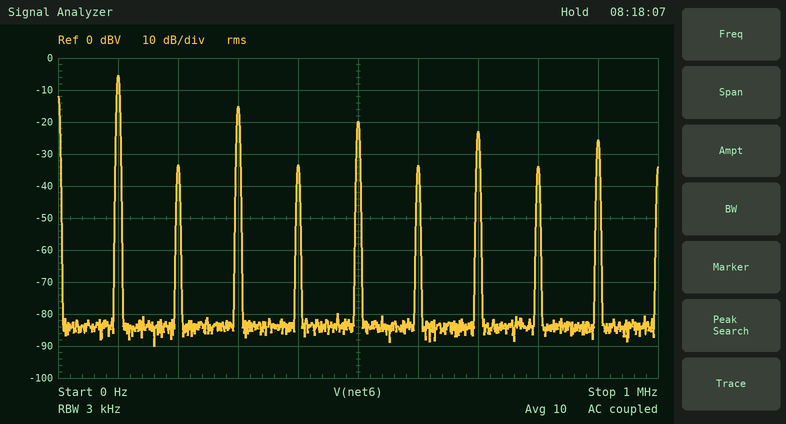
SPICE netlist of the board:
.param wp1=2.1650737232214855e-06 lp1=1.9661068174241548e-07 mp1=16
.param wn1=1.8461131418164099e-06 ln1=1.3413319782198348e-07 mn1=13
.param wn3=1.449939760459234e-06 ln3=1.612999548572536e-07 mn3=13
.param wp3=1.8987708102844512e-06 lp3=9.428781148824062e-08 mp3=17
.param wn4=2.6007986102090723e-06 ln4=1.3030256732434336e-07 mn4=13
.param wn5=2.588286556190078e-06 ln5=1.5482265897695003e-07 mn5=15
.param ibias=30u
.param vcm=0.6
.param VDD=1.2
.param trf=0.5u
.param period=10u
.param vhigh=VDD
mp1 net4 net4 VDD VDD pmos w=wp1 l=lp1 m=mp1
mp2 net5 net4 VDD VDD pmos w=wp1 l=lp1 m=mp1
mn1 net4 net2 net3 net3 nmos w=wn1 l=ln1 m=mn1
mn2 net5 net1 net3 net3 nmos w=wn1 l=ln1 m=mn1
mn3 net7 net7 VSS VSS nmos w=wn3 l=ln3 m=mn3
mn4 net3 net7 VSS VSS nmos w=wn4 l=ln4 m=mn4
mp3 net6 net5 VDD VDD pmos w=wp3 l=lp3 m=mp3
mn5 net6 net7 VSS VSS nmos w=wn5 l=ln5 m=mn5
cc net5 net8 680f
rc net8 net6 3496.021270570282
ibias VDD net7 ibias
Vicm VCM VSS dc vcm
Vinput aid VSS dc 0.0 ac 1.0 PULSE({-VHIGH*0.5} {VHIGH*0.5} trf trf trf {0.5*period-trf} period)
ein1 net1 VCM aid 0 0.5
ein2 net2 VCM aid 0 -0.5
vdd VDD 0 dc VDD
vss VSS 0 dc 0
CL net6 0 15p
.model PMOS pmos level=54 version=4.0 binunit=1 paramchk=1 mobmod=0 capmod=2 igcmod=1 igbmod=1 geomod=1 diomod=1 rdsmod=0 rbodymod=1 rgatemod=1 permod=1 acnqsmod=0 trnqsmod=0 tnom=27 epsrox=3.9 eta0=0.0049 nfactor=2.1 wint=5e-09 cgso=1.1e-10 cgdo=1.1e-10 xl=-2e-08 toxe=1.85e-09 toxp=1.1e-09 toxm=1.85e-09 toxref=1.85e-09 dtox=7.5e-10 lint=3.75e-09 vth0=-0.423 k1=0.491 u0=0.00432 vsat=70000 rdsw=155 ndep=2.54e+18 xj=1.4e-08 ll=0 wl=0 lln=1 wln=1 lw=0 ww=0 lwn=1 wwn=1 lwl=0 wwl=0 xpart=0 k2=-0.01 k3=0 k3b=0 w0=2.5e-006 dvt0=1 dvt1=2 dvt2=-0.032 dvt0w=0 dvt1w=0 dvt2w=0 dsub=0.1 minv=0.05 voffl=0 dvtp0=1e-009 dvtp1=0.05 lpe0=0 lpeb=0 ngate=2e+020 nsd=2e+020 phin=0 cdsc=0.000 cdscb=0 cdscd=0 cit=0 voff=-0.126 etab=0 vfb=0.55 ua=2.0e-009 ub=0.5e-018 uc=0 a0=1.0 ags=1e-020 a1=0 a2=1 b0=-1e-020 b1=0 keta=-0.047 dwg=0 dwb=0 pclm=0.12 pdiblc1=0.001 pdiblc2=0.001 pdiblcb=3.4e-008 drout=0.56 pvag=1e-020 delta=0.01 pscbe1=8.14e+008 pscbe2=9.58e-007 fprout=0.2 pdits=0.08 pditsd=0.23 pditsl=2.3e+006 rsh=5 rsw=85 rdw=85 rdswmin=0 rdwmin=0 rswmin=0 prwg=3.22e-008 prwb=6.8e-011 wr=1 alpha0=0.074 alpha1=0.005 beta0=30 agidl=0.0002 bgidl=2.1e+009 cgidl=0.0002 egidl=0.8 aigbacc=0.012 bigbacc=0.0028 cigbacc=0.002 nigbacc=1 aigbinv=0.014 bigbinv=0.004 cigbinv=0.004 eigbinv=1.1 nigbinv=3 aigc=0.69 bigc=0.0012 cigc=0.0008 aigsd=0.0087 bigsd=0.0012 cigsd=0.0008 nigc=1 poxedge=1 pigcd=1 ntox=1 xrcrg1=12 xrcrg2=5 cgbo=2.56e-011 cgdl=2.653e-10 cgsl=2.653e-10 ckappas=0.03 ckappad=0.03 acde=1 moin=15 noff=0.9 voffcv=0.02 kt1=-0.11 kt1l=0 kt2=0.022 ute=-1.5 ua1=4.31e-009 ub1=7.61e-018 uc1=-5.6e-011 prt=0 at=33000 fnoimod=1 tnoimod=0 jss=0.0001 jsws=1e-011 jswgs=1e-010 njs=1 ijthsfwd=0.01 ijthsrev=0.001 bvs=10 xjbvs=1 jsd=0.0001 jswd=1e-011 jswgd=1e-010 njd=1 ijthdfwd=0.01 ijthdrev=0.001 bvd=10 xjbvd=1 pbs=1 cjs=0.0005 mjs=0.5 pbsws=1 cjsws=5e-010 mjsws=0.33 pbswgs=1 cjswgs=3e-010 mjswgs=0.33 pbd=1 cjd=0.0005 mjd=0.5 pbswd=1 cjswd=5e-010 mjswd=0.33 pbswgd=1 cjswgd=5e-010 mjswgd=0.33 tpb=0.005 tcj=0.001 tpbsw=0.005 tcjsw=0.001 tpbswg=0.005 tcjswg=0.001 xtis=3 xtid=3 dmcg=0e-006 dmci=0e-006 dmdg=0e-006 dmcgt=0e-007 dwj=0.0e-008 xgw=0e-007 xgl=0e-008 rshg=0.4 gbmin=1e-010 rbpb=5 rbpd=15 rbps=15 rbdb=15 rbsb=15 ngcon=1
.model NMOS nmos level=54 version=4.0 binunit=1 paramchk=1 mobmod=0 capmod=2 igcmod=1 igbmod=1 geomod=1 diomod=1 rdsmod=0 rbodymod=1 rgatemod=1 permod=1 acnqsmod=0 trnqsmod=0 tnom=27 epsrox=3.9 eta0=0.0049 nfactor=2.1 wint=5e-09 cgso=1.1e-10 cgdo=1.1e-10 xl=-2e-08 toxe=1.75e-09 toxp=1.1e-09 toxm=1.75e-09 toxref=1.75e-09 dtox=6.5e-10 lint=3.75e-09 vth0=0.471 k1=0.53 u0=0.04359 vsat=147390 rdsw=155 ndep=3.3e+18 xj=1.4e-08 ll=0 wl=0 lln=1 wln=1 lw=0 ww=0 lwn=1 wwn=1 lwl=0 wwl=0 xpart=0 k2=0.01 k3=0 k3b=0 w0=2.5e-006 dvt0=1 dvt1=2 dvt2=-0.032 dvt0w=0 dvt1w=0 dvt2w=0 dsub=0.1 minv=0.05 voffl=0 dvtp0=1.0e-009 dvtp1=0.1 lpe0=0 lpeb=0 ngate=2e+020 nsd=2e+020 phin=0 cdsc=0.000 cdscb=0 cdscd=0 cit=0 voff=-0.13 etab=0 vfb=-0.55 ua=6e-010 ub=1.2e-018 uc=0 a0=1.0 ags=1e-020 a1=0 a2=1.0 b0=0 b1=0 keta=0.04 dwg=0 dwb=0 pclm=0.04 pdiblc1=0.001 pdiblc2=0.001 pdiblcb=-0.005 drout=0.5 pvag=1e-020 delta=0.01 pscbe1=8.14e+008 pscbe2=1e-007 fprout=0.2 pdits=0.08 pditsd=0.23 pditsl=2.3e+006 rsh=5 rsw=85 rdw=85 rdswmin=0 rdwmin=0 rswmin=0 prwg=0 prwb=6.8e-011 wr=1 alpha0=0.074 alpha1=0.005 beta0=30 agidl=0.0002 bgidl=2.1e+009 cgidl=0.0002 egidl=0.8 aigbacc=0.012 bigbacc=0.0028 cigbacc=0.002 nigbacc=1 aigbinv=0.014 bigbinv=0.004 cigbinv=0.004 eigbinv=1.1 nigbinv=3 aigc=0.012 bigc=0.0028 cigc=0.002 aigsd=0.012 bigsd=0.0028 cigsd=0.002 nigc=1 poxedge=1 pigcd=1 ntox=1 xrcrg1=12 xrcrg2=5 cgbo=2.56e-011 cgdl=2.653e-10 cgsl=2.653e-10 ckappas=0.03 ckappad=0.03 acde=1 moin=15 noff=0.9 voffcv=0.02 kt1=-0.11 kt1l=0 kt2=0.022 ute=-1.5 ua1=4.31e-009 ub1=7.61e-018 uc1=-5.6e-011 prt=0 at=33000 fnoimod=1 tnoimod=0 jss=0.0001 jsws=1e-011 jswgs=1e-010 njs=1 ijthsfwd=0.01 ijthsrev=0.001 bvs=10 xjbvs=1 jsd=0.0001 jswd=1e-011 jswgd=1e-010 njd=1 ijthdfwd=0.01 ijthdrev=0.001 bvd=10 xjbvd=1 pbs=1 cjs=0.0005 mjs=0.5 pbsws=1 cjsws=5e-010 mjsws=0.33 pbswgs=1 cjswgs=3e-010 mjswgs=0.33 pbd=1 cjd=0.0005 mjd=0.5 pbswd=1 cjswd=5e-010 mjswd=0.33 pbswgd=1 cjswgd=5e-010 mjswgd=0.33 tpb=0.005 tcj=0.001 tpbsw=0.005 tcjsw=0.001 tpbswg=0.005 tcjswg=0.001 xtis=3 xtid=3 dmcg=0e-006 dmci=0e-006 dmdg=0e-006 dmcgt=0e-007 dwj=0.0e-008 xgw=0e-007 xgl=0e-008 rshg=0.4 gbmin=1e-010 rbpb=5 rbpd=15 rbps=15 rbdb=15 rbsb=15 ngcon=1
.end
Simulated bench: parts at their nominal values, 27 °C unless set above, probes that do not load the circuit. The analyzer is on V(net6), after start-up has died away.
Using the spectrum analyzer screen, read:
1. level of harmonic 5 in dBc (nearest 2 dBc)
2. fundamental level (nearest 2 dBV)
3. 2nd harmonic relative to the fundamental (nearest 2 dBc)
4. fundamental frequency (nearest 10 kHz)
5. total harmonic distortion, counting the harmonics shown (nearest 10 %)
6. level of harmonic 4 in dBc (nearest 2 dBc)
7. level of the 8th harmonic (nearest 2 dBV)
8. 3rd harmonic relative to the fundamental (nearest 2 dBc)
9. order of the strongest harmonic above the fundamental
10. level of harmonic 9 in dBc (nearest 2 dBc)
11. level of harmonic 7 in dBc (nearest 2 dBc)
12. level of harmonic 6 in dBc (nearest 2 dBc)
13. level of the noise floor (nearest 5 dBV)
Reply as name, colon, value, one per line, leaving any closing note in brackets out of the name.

level of harmonic 5 in dBc: -14 dBc
fundamental level: -6 dBV
2nd harmonic relative to the fundamental: -28 dBc
fundamental frequency: 100 kHz
total harmonic distortion, counting the harmonics shown: 40 %
level of harmonic 4 in dBc: -28 dBc
level of the 8th harmonic: -34 dBV
3rd harmonic relative to the fundamental: -10 dBc
order of the strongest harmonic above the fundamental: 3
level of harmonic 9 in dBc: -20 dBc
level of harmonic 7 in dBc: -18 dBc
level of harmonic 6 in dBc: -28 dBc
level of the noise floor: -85 dBV
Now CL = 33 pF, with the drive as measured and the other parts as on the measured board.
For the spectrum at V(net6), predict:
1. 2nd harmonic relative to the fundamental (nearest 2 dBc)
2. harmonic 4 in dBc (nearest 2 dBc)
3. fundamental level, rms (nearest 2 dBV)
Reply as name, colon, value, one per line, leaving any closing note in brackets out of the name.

2nd harmonic relative to the fundamental: -22 dBc
harmonic 4 in dBc: -22 dBc
fundamental level, rms: -6 dBV
